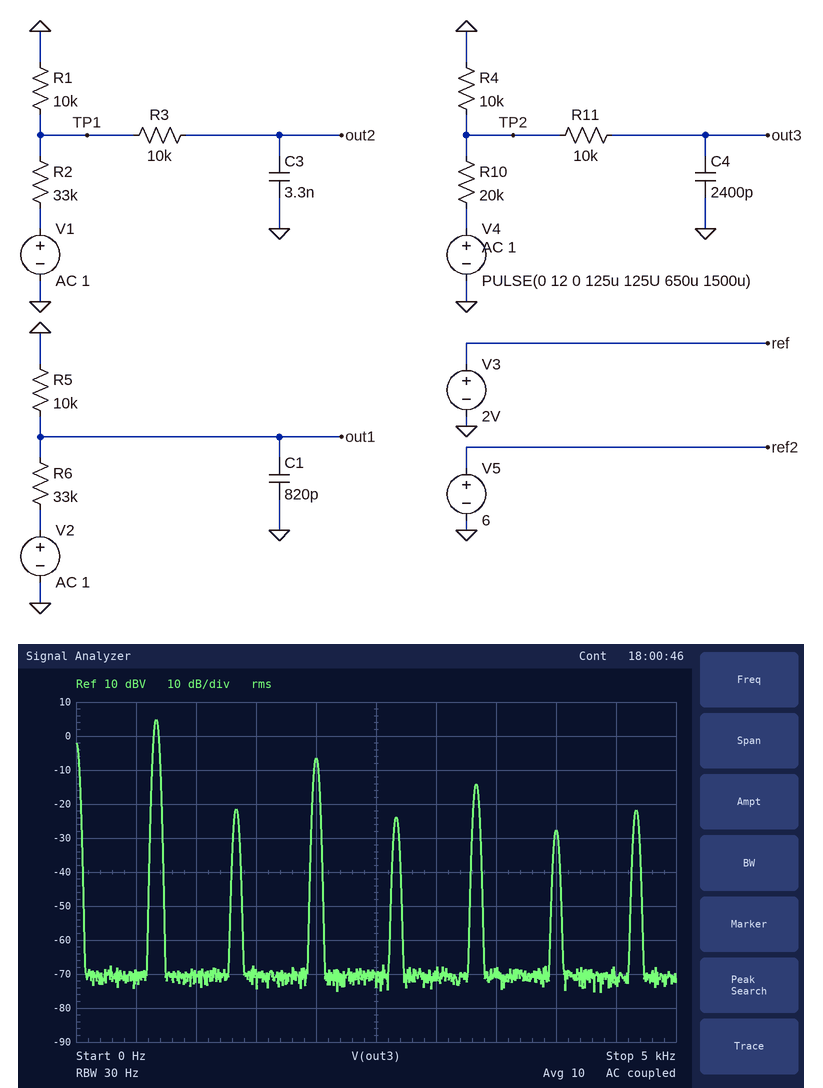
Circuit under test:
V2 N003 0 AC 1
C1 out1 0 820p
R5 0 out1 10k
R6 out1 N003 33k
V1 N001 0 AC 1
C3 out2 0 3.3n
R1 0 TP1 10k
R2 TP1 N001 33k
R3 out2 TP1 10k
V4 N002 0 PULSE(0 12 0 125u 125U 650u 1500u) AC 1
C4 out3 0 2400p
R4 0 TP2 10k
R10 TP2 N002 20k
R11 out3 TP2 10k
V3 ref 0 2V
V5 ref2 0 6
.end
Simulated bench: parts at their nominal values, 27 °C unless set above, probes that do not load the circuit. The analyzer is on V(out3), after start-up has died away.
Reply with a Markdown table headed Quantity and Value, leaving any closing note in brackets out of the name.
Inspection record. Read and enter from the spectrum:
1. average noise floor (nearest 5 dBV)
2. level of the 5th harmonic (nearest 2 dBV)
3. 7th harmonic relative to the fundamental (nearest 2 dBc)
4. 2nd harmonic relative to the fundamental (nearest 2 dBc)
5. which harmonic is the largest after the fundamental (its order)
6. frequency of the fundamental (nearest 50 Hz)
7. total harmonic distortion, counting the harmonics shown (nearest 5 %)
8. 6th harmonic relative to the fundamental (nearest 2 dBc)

| Quantity | Value |
|---|---|
| average noise floor | -70 dBV |
| level of the 5th harmonic | -14 dBV |
| 7th harmonic relative to the fundamental | -26 dBc |
| 2nd harmonic relative to the fundamental | -26 dBc |
| which harmonic is the largest after the fundamental | 3 |
| frequency of the fundamental | 650 Hz |
| total harmonic distortion, counting the harmonics shown | 30 % |
| 6th harmonic relative to the fundamental | -32 dBc |
